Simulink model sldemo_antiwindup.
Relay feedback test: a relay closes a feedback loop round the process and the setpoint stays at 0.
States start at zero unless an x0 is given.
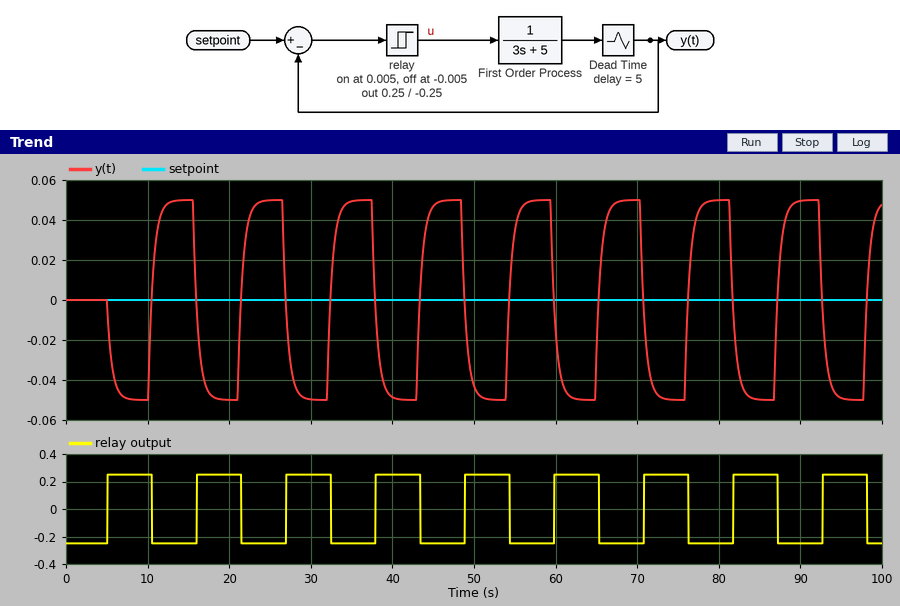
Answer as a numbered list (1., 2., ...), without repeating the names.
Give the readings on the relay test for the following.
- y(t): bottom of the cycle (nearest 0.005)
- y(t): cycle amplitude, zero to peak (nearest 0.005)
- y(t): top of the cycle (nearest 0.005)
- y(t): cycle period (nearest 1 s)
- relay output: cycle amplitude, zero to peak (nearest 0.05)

1. -0.050
2. 0.050
3. 0.050
4. 11 s
5. 0.25
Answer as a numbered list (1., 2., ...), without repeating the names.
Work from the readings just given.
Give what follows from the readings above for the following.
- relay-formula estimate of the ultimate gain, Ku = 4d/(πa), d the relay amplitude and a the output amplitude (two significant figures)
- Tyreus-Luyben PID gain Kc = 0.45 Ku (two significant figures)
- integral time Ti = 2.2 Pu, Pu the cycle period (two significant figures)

1. 6.4
2. 2.9
3. 24 s
